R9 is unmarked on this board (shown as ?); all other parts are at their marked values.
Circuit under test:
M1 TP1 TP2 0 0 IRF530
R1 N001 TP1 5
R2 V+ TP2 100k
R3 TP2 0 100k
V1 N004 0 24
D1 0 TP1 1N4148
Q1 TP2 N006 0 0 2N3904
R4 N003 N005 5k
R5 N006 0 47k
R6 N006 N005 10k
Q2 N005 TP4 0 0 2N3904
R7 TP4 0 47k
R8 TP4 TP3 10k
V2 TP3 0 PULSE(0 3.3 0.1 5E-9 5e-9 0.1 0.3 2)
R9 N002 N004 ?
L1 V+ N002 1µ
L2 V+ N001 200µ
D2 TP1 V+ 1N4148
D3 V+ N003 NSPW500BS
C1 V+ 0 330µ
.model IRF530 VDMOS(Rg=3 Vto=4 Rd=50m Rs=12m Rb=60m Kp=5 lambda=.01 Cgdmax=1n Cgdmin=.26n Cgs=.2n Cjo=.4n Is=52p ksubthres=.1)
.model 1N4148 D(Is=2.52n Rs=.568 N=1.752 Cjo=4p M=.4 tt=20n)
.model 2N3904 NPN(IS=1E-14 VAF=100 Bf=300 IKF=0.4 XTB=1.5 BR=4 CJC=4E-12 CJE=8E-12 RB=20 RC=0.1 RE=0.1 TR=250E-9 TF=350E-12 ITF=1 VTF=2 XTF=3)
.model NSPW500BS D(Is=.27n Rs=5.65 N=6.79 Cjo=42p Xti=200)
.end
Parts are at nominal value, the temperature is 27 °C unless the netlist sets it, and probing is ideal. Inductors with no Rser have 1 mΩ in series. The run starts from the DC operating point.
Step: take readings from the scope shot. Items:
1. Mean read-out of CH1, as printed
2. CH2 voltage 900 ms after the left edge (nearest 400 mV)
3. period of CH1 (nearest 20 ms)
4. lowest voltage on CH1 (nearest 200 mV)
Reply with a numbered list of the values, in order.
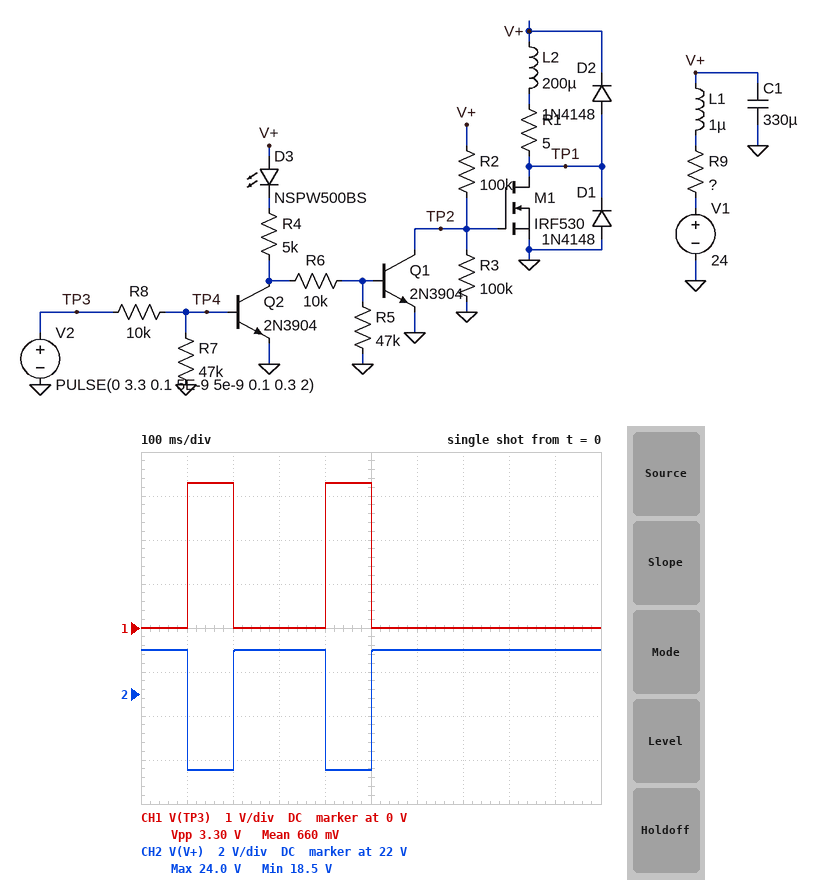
1. 660 mV
2. 24.0 V
3. 300 ms
4. 0 V
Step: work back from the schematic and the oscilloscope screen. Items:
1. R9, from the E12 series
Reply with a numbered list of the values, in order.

1. 1.5 Ω
